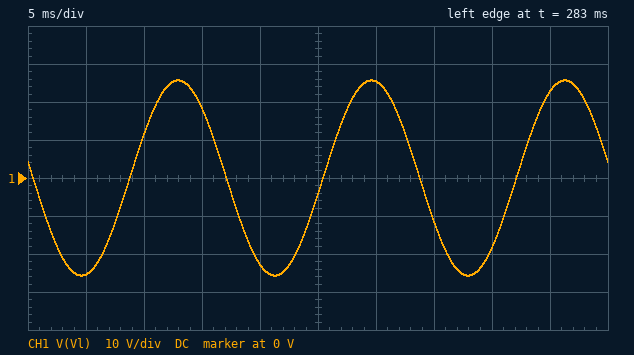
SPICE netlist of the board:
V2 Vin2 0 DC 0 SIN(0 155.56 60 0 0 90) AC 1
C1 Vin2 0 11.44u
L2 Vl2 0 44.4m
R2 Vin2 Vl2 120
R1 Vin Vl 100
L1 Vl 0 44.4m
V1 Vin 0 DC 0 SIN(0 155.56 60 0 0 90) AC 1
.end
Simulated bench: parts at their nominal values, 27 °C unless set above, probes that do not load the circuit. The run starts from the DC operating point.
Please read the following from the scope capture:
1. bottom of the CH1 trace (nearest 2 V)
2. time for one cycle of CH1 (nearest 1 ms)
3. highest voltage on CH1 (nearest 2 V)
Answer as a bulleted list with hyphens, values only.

- -26 V
- 17 ms
- 26 V
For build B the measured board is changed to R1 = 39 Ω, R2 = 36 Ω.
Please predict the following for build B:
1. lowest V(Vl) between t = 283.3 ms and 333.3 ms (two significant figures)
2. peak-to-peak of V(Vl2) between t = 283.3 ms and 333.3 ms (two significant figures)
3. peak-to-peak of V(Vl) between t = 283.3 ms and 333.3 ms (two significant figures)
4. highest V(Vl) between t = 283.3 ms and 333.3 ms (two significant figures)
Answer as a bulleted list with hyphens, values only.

- -61 V
- 130 V
- 120 V
- 61 V
